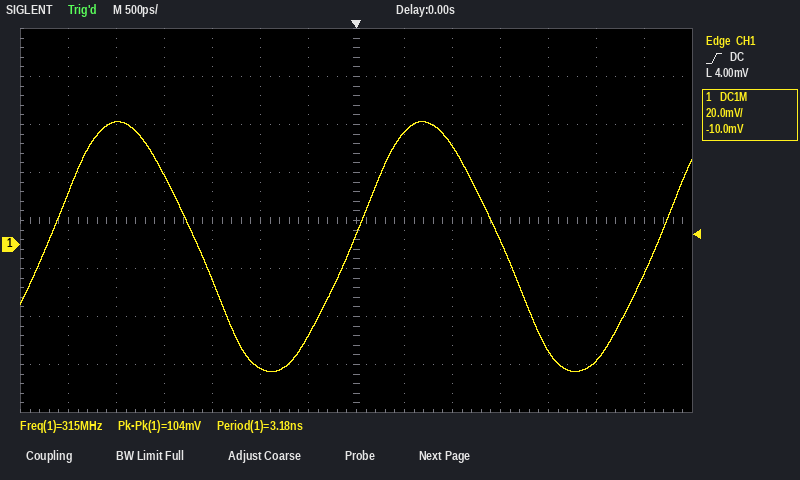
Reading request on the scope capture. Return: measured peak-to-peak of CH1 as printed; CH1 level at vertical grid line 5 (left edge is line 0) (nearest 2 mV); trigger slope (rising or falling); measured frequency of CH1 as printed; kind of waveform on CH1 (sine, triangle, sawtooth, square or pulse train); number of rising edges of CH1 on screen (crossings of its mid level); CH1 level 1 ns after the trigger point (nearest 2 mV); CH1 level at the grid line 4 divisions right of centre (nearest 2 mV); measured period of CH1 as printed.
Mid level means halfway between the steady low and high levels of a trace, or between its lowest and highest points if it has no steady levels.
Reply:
104 mV
-52 mV
rising
315 MHz
sine
3
42 mV
-44 mV
3.18 ns
